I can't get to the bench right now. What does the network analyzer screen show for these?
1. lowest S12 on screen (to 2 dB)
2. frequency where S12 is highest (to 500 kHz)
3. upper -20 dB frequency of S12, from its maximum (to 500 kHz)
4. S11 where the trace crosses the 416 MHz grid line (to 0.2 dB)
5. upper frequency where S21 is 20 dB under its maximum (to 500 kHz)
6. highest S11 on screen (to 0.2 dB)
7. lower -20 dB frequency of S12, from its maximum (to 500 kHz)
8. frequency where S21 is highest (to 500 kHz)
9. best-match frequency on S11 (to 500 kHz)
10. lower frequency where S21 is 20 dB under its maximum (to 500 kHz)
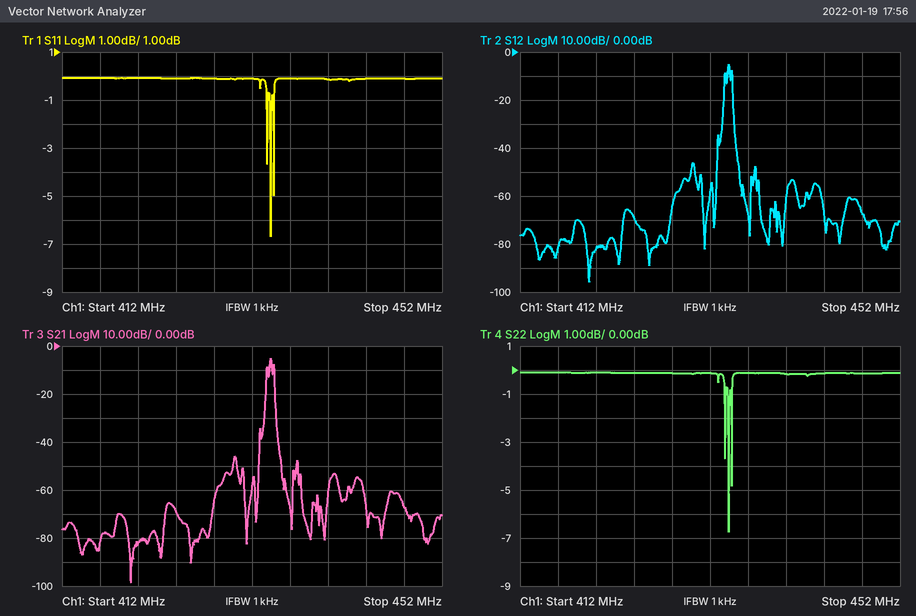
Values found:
-96 dB
434.0 MHz
434.5 MHz
0.0 dB
434.5 MHz
0.0 dB
433.5 MHz
434.0 MHz
434.0 MHz
433.5 MHz
